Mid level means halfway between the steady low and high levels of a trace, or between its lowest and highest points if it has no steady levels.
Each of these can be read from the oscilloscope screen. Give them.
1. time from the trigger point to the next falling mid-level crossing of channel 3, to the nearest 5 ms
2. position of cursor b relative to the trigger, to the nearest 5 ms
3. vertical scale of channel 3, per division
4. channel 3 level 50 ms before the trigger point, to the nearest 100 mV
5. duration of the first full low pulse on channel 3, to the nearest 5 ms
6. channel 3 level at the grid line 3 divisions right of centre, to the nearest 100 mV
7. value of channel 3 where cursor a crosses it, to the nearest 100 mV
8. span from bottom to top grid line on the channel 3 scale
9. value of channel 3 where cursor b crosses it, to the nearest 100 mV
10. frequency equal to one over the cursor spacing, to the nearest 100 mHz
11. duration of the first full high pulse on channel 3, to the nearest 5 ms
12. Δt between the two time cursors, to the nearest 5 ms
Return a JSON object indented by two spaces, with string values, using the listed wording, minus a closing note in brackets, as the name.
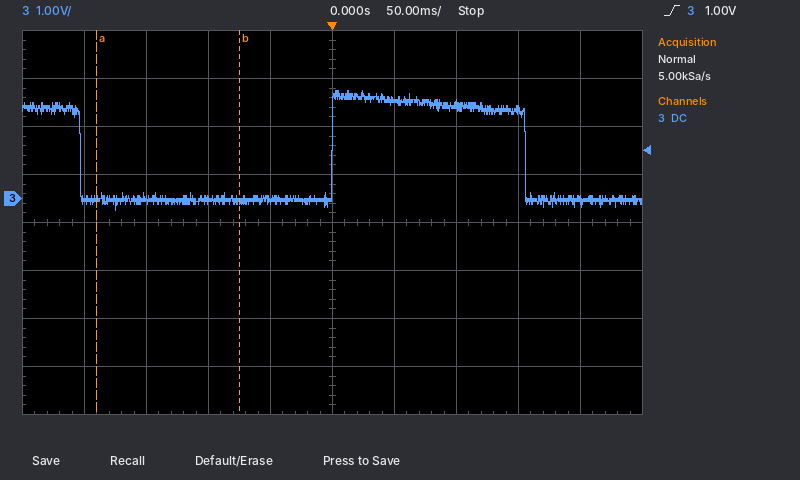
{
  "time from the trigger point to the next falling mid-level crossing of channel 3, to the nearest 5 ms": "155 ms",
  "position of cursor b relative to the trigger, to the nearest 5 ms": "-75 ms",
  "vertical scale of channel 3, per division": "1 V",
  "channel 3 level 50 ms before the trigger point, to the nearest 100 mV": "0.0 V",
  "duration of the first full low pulse on channel 3, to the nearest 5 ms": "205 ms",
  "channel 3 level at the grid line 3 divisions right of centre, to the nearest 100 mV": "1.8 V",
  "value of channel 3 where cursor a crosses it, to the nearest 100 mV": "0.0 V",
  "span from bottom to top grid line on the channel 3 scale": "8 V",
  "value of channel 3 where cursor b crosses it, to the nearest 100 mV": "0.0 V",
  "frequency equal to one over the cursor spacing, to the nearest 100 mHz": "8.7 Hz",
  "duration of the first full high pulse on channel 3, to the nearest 5 ms": "155 ms",
  "Δt between the two time cursors, to the nearest 5 ms": "115 ms"
}
